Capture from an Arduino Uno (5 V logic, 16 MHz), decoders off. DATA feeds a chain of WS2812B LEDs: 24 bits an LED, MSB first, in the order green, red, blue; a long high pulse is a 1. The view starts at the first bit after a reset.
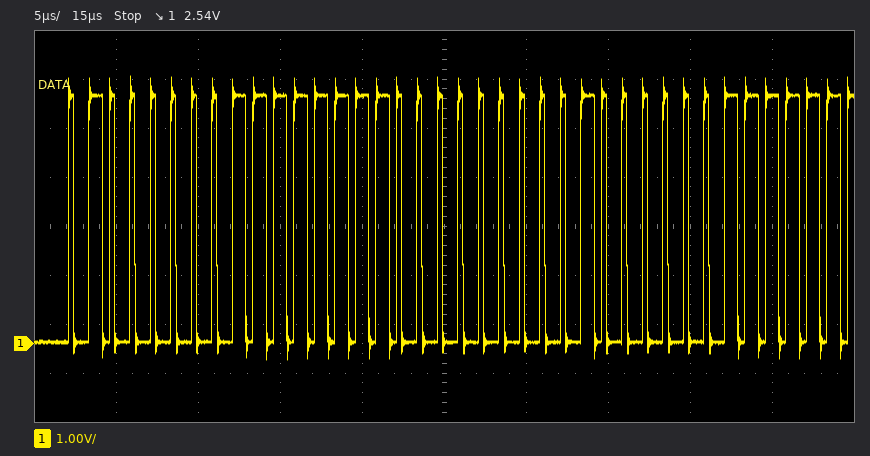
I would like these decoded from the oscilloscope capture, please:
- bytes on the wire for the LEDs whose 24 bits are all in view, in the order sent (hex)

40 FF 00
